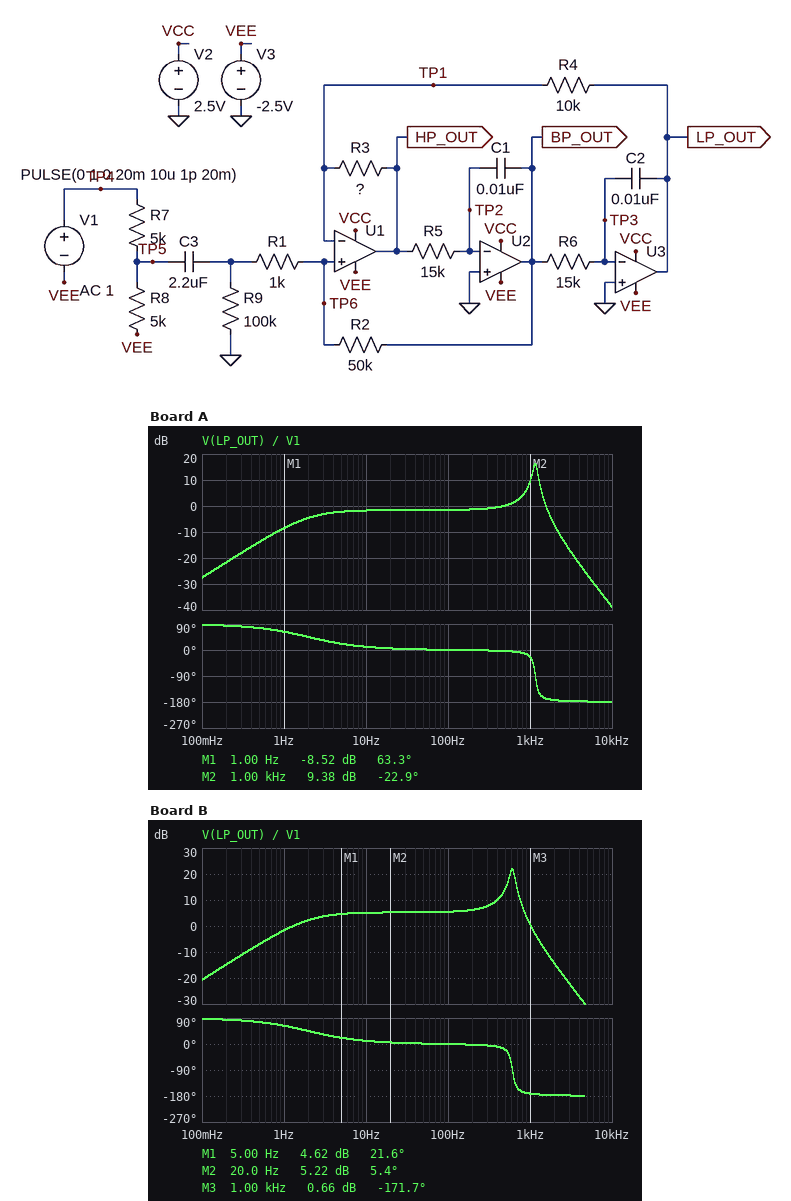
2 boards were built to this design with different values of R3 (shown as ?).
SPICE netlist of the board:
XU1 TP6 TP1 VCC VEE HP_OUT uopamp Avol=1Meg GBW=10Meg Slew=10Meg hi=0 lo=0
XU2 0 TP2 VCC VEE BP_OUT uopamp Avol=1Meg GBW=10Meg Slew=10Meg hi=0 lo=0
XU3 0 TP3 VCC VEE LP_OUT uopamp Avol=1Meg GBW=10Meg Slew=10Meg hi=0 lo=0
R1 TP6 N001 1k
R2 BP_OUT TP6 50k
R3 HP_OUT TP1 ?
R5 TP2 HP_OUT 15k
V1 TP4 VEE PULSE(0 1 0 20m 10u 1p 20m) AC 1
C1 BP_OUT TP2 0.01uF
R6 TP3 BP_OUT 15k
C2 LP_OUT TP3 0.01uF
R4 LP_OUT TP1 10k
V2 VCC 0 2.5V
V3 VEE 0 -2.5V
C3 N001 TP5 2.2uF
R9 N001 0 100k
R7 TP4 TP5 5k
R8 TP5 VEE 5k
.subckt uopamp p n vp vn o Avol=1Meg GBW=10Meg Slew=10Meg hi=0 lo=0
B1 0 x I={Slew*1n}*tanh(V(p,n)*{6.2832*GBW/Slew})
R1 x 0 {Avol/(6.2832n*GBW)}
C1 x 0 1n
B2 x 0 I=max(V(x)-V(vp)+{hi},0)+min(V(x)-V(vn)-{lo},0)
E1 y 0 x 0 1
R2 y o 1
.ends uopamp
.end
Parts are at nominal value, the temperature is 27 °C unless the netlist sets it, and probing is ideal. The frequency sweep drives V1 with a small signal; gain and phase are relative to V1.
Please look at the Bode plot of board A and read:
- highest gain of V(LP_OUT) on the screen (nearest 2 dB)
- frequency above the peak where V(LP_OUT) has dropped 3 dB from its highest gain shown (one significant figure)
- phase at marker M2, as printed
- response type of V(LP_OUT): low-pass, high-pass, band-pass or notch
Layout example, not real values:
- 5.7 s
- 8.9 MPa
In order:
- 16 dB
- 1 kHz
- -22.9 deg
- band-pass
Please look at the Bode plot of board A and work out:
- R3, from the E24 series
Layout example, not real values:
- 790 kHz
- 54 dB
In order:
- 12 kΩ
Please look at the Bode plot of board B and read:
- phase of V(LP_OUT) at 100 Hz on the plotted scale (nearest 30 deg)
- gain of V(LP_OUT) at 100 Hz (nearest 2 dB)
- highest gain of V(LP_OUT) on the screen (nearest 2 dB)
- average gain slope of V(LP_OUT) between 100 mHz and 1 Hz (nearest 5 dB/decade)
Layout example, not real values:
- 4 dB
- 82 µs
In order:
- 0 deg
- 6 dB
- 22 dB
- 20 dB/decade
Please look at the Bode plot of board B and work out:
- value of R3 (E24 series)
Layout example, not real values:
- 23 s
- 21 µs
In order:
- 3.3 kΩ
